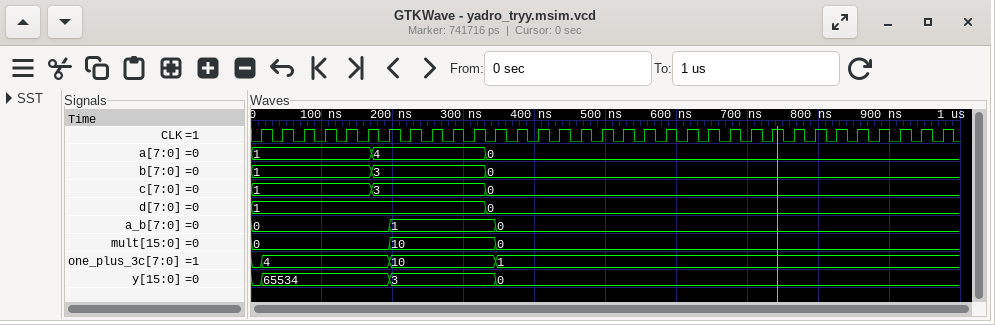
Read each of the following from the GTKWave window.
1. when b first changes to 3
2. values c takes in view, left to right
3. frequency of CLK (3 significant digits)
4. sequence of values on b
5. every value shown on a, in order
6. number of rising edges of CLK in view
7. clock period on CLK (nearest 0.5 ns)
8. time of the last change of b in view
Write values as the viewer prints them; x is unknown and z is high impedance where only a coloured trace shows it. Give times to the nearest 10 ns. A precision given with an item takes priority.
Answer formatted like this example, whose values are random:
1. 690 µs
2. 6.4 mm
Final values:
1. 170 ns
2. 1, 3, 0
3. 33.3 MHz
4. 1, 3, 0
5. 1, 4, 0
6. 33
7. 30 ns
8. 330 ns
